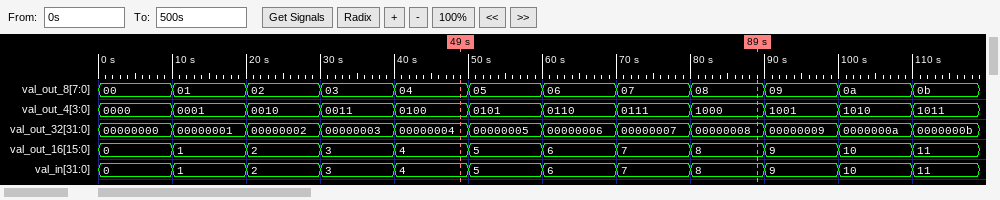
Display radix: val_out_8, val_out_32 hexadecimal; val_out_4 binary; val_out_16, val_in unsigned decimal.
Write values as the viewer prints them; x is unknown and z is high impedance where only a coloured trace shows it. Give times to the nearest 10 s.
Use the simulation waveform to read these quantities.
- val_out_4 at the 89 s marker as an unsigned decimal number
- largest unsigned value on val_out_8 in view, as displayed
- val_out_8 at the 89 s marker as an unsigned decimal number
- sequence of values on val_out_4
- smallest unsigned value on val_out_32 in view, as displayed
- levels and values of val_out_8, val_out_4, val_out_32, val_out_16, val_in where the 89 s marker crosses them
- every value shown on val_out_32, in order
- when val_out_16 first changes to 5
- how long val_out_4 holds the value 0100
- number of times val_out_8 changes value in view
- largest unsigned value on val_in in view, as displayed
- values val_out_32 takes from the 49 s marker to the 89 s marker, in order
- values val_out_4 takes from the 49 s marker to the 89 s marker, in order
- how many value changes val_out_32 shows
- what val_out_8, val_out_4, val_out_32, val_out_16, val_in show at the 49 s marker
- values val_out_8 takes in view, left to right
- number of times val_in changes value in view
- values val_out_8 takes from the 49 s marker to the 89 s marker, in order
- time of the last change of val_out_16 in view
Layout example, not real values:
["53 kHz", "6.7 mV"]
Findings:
["8", "0b", "8", "0000, 0001, 0010, 0011, 0100, 0101, 0110, 0111, 1000, 1001, 1010, 1011", "00000000", "val_out_8=08, val_out_4=1000, val_out_32=00000008, val_out_16=8, val_in=8", "00000000, 00000001, 00000002, 00000003, 00000004, 00000005, 00000006, 00000007, 00000008, 00000009, 0000000a, 0000000b", "50 s", "10 s", "11", "11", "00000004, 00000005, 00000006, 00000007, 00000008", "0100, 0101, 0110, 0111, 1000", "11", "val_out_8=04, val_out_4=0100, val_out_32=00000004, val_out_16=4, val_in=4", "00, 01, 02, 03, 04, 05, 06, 07, 08, 09, 0a, 0b", "11", "04, 05, 06, 07, 08", "110 s"]
